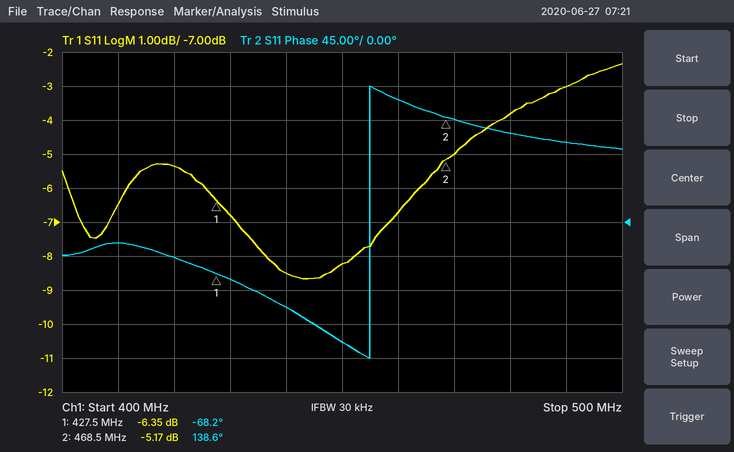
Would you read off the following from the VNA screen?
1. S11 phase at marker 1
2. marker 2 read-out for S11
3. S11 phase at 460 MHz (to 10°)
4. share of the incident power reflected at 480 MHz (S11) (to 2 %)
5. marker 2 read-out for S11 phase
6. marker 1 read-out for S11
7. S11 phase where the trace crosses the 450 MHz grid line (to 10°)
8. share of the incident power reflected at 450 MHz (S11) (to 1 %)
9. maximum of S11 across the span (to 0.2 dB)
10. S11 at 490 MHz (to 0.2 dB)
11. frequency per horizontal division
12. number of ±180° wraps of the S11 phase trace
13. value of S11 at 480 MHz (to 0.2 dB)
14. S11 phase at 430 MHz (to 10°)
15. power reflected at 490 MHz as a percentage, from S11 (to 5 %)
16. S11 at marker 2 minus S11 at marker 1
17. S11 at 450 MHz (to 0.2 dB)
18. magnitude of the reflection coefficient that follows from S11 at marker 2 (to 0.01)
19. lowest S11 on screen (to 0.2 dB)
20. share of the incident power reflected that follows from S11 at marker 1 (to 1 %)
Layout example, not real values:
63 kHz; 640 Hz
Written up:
-68.2°; -5.17 dB; 160°; 42 %; 138.6°; -6.35 dB; -160°; 15 %; -2.4 dB; -3.0 dB; 10 MHz; 1; -3.8 dB; -80°; 50 %; 1.18 dB; -8.2 dB; 0.55; -8.6 dB; 23 %
